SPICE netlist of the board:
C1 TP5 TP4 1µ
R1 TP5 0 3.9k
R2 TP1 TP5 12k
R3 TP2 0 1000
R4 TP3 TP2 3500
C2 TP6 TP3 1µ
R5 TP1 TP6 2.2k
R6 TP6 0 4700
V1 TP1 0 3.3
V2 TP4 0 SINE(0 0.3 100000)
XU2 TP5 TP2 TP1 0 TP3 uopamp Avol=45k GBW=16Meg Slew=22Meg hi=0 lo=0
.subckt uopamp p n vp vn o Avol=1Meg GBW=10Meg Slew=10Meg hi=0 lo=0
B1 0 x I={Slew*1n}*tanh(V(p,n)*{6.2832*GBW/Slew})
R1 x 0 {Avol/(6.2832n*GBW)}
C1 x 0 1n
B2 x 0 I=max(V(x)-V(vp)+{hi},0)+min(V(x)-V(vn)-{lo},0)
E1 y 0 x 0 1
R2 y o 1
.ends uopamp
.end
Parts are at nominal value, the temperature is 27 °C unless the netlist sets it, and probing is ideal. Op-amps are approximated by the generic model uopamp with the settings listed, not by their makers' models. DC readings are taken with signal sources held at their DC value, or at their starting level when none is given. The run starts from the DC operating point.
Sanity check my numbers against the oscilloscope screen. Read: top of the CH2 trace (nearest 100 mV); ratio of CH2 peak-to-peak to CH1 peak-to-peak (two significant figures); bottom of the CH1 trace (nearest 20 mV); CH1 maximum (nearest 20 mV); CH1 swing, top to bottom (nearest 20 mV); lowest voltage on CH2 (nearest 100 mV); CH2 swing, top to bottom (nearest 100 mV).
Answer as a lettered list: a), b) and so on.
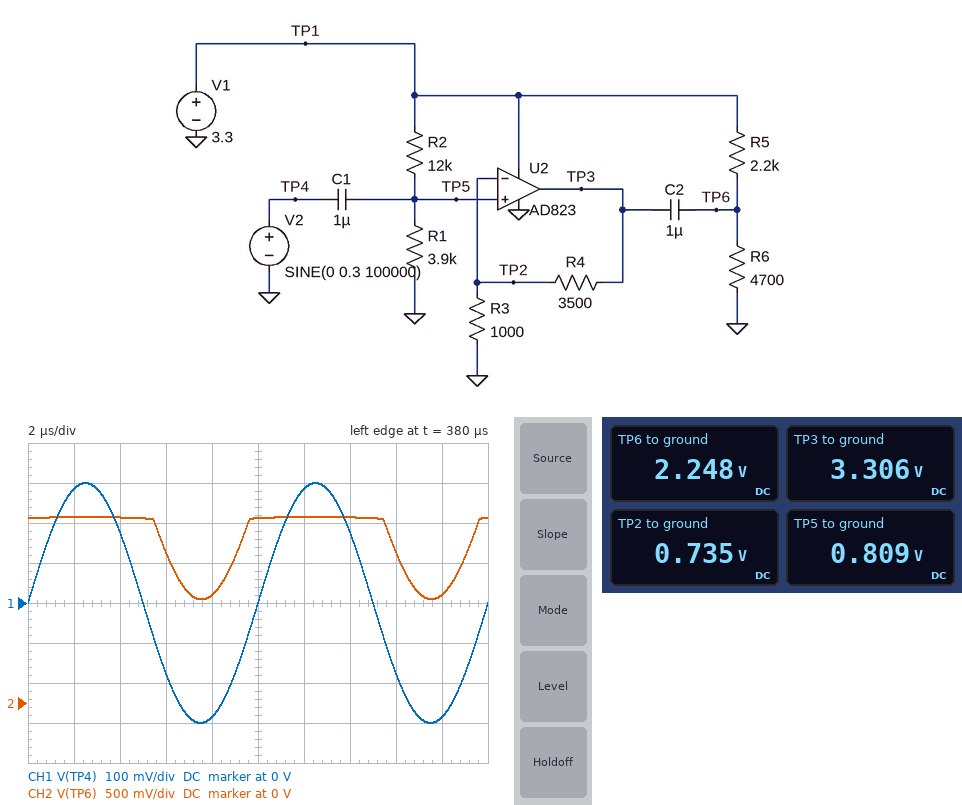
a) 2.3 V
b) 1.7
c) -300 mV
d) 300 mV
e) 600 mV
f) 1.3 V
g) 1.0 V
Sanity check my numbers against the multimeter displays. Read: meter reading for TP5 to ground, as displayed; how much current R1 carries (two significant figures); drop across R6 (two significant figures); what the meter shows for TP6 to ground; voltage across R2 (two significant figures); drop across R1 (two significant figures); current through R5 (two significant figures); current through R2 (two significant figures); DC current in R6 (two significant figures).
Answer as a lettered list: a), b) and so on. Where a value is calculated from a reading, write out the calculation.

a) 0.809 V
b) (809 mV) / 3.9 kΩ = 210 µA
c) 2.248 V = 2.2 V
d) 2.248 V
e) 3.3 V - 809 mV = 2.5 V
f) 809 mV = 810 mV
g) (3.3 V - 2.248 V) / 2.2 kΩ = 480 µA
h) (3.3 V - 809 mV) / 12 kΩ = 210 µA
i) (2.248 V) / 4.7 kΩ = 480 µA
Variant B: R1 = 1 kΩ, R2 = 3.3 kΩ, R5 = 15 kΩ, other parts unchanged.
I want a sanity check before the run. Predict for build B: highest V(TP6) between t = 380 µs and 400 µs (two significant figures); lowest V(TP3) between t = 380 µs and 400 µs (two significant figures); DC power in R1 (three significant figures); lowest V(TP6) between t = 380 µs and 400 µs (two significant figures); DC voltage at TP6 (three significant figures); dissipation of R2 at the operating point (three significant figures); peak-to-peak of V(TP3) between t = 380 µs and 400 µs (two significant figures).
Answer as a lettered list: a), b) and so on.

a) 840 mV
b) 2.1 V
c) 589 µW
d) -380 mV
e) 787 mV
f) 1.94 mW
g) 1.2 V
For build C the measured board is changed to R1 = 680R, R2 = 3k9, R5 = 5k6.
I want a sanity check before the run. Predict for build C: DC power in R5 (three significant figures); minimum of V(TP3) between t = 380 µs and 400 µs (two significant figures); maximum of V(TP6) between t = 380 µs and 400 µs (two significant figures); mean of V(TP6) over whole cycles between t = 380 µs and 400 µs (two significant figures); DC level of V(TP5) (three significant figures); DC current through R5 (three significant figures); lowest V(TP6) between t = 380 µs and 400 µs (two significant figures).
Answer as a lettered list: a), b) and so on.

a) 575 µW
b) 850 mV
c) 2.6 V
d) 1.5 V
e) 490 mV
f) 320 µA
g) 160 mV
